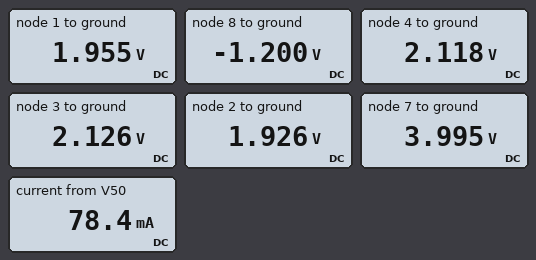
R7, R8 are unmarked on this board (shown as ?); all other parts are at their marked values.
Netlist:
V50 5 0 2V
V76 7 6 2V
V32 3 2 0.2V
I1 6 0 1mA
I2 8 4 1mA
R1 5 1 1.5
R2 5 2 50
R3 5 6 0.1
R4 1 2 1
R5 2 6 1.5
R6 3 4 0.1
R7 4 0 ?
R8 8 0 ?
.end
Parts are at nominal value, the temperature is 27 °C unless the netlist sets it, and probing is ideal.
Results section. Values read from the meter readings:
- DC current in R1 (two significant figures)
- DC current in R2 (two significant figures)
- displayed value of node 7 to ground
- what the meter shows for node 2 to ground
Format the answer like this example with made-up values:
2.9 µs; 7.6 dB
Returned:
30 mA; 1.5 mA; 3.995 V; 1.926 V
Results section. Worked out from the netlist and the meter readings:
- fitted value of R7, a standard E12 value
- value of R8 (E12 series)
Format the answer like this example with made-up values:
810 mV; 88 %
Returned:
27 Ω; 1.2 kΩ
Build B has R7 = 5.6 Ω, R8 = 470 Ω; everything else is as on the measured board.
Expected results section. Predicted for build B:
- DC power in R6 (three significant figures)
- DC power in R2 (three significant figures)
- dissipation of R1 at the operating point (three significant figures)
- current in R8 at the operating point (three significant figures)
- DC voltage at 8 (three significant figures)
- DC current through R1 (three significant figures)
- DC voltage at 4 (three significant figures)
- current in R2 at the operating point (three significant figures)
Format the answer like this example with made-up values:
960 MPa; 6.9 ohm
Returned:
10.9 mW; 1.99 mW; 23.9 mW; 1.00 mA; -470 mV; 126 mA; 1.85 V; 6.31 mA
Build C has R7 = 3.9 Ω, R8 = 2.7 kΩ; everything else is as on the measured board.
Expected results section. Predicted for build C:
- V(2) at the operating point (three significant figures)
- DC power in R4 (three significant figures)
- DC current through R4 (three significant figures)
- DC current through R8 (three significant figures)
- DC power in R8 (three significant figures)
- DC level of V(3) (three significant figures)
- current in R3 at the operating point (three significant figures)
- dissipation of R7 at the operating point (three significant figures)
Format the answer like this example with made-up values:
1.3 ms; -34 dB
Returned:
1.58 V; 28.8 mW; 170 mA; 1.00 mA; 2.70 mW; 1.78 V; 266 mA; 769 mW
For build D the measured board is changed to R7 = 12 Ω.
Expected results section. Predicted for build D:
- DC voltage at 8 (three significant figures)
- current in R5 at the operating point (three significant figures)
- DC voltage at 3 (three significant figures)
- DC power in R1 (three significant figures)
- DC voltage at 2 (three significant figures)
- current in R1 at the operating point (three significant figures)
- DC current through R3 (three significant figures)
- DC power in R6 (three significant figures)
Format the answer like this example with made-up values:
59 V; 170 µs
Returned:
-1.20 V; 100 mA; 2.04 V; 6.18 mW; 1.84 V; 64.2 mA; 101 mA; 2.81 mW
